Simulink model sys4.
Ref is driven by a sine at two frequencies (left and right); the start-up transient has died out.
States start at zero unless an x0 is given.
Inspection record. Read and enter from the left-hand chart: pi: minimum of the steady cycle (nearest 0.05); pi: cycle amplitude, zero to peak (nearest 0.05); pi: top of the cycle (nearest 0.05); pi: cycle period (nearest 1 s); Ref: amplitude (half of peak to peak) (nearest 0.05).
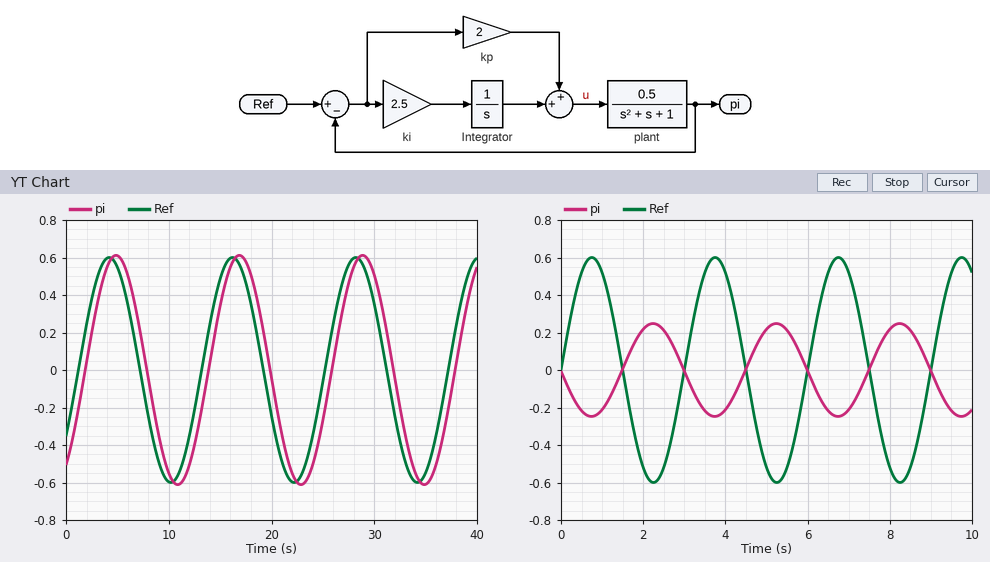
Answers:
-0.60
0.60
0.60
12 s
0.60
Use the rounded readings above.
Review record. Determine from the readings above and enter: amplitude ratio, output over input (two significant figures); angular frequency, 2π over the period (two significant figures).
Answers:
1.0
0.52 rad/s
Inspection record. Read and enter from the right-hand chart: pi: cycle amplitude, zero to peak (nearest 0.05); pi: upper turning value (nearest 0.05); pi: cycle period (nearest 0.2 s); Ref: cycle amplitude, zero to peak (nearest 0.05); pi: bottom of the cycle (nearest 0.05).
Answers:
0.25
0.25
3.0 s
0.60
-0.25
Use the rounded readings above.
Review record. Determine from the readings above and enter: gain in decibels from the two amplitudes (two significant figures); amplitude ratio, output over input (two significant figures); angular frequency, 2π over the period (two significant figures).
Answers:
-7.6 dB
0.42
2.1 rad/s
